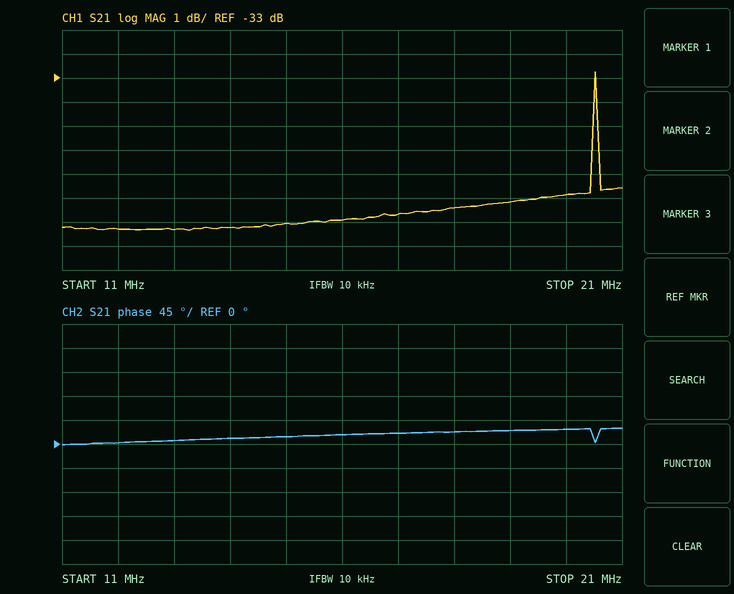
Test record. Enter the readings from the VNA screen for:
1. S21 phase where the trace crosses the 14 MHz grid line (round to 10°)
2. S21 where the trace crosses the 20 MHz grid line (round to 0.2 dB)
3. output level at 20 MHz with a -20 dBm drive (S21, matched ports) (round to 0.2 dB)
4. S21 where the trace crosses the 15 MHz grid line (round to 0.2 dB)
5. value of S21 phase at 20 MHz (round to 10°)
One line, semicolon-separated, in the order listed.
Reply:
10°; -37.8 dB; -57.8 dBm; -39.0 dB; 30°
